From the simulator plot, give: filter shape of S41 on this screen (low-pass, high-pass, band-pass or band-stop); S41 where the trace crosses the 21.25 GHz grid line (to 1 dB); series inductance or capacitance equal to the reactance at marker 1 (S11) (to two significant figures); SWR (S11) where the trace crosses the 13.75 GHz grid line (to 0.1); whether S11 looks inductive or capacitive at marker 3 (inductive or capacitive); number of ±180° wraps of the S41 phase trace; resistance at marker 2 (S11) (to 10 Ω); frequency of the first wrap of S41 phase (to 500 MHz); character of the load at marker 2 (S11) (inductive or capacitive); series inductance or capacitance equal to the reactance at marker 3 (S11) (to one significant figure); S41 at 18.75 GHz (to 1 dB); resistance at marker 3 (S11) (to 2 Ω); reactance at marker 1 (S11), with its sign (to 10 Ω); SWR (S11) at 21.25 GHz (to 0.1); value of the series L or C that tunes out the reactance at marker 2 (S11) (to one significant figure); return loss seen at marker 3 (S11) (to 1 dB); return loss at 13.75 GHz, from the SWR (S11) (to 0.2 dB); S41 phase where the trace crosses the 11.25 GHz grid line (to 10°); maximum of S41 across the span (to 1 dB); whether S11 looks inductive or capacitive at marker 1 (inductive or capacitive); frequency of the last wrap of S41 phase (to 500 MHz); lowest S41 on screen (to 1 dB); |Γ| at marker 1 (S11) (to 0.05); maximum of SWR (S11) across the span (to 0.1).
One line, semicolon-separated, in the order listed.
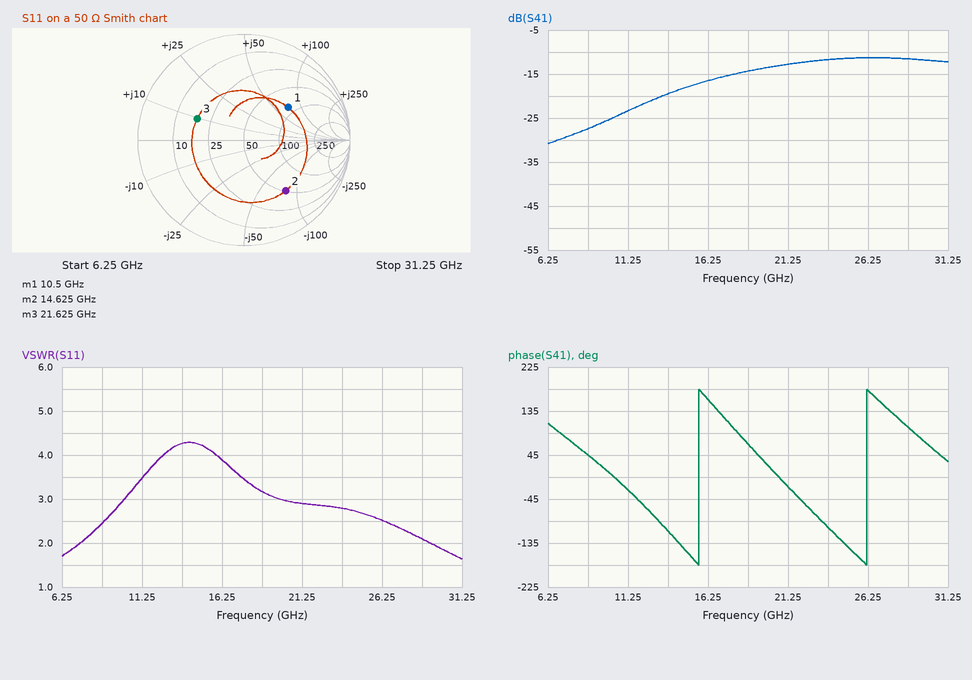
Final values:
high-pass; -13 dB; 1.1 nH; 4.3; inductive; 2; 50 Ω; 15.5 GHz; capacitive; 70 pH; -14 dB; 18 Ω; +70 Ω; 2.9; 900 pH; 6 dB; 4.2 dB; -30°; -11 dB; inductive; 26.0 GHz; -31 dB; 0.50; 4.3
